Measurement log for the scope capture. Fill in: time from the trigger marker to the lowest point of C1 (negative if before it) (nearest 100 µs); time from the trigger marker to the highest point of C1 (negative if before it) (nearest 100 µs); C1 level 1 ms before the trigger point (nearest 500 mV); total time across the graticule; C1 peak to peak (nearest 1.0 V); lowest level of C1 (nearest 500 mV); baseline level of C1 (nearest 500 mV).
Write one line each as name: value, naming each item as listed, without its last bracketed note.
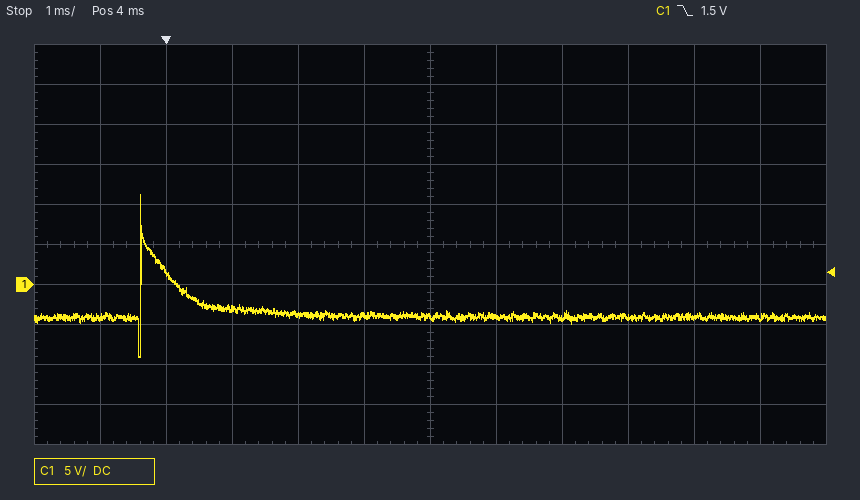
time from the trigger marker to the lowest point of C1 (negative if before it): -400 µs
time from the trigger marker to the highest point of C1 (negative if before it): -400 µs
C1 level 1 ms before the trigger point: -4.0 V
total time across the graticule: 12 ms
C1 peak to peak: 20.0 V
lowest level of C1: -9.0 V
baseline level of C1: -4.0 V
